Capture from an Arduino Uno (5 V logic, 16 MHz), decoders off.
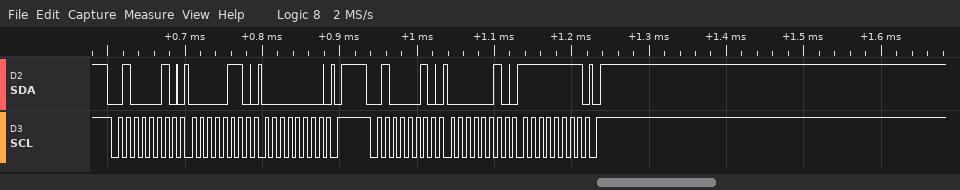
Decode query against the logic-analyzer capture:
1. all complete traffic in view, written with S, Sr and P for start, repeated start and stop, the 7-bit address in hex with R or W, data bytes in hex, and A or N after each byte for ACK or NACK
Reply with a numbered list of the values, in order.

1. S 21W A 06 A 00 A P S 21W A 02 A FF A P
